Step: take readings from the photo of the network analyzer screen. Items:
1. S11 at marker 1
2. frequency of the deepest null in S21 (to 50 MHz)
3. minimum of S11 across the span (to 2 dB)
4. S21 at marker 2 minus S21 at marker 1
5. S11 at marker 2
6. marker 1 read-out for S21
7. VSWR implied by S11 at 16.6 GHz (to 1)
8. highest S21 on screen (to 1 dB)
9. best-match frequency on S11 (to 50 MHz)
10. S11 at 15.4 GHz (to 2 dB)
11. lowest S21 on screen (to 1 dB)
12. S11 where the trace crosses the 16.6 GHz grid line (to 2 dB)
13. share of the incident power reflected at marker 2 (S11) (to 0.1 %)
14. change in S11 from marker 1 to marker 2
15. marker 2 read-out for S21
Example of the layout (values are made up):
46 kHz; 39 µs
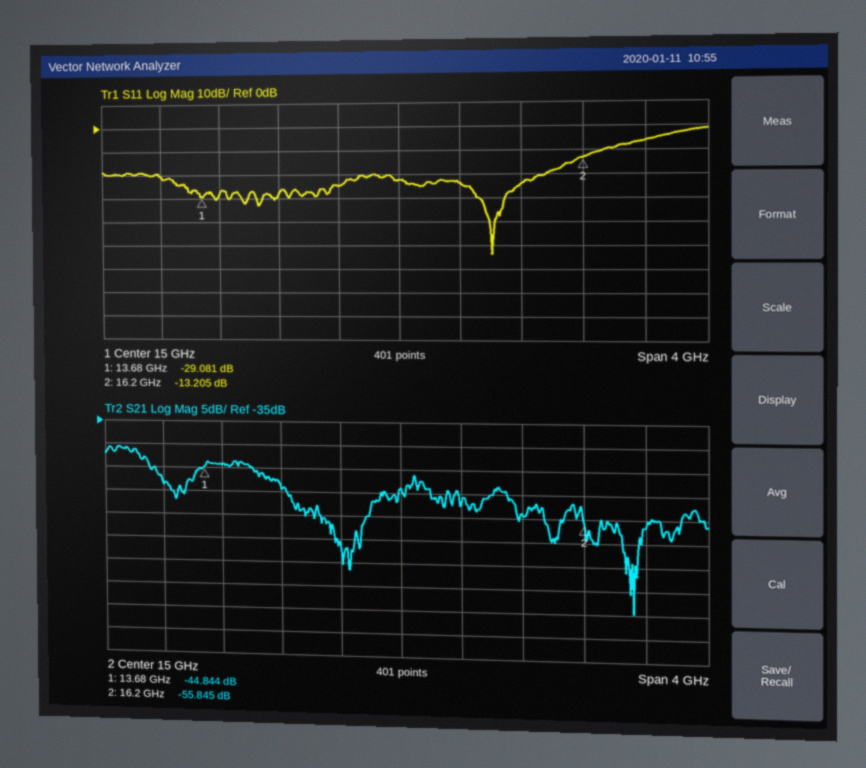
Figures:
-29.081 dB; 16.50 GHz; -54 dB; -11.001 dB; -13.205 dB; -44.844 dB; 3; -41 dB; 15.60 GHz; -24 dB; -75 dB; -6 dB; 4.8 %; 15.876 dB; -55.845 dB
